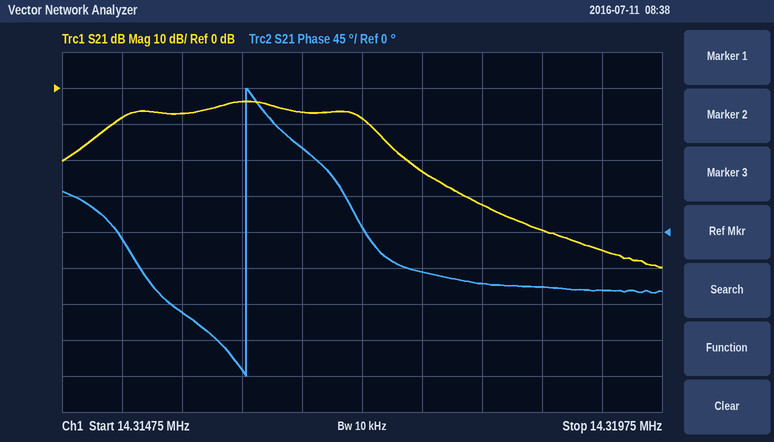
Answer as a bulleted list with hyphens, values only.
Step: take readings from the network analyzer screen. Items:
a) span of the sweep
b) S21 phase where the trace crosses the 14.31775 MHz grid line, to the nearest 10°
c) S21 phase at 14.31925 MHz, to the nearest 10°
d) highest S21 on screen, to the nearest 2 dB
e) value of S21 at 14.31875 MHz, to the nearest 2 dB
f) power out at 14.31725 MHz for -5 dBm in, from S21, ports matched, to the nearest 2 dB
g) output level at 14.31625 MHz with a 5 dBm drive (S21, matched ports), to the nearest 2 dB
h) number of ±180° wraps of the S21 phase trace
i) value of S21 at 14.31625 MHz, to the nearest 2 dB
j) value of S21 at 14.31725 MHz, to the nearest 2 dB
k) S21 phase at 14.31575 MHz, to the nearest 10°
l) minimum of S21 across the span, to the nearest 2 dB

- 5 kHz
- -50°
- -70°
- -4 dB
- -40 dB
- -14 dBm
- 2 dBm
- 1
- -4 dB
- -8 dB
- -100°
- -50 dB
